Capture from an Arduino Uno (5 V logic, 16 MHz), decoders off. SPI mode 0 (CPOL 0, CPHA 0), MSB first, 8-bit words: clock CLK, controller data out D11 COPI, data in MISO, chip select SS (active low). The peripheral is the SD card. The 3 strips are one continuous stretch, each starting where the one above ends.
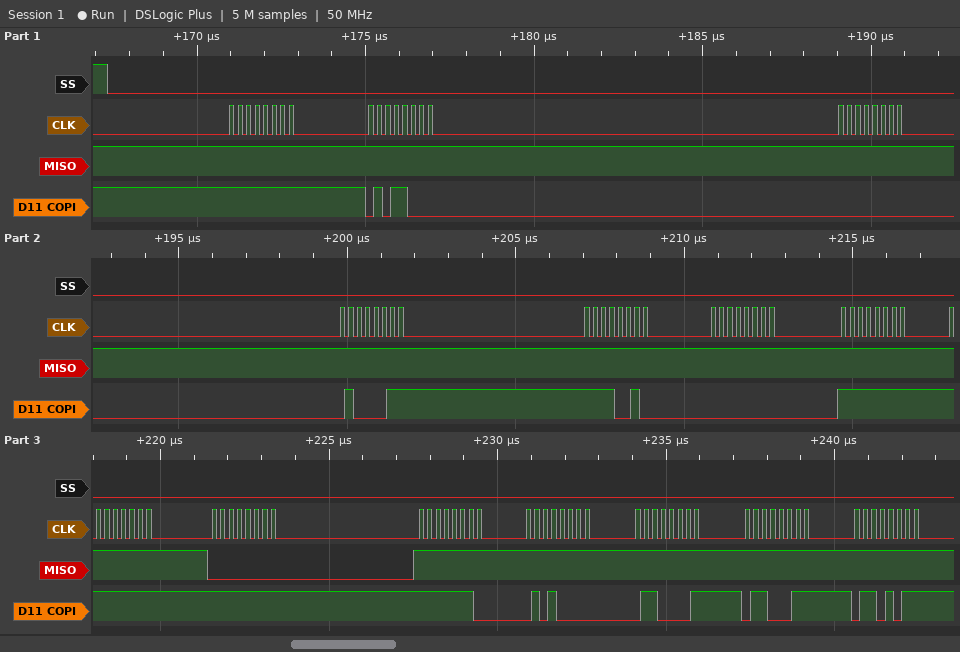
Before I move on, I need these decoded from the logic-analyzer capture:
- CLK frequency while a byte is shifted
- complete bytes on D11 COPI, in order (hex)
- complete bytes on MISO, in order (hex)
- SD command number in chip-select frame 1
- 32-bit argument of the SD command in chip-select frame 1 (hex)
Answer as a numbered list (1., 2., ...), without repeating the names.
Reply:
1. 4 MHz
2. FF 58 00 43 F2 00 FF FF FF FE 50 61 63 6B
3. FF FF FF FF FF FF FF FF 00 FF FF FF FF FF
4. CMD24
5. 0x0043F200
